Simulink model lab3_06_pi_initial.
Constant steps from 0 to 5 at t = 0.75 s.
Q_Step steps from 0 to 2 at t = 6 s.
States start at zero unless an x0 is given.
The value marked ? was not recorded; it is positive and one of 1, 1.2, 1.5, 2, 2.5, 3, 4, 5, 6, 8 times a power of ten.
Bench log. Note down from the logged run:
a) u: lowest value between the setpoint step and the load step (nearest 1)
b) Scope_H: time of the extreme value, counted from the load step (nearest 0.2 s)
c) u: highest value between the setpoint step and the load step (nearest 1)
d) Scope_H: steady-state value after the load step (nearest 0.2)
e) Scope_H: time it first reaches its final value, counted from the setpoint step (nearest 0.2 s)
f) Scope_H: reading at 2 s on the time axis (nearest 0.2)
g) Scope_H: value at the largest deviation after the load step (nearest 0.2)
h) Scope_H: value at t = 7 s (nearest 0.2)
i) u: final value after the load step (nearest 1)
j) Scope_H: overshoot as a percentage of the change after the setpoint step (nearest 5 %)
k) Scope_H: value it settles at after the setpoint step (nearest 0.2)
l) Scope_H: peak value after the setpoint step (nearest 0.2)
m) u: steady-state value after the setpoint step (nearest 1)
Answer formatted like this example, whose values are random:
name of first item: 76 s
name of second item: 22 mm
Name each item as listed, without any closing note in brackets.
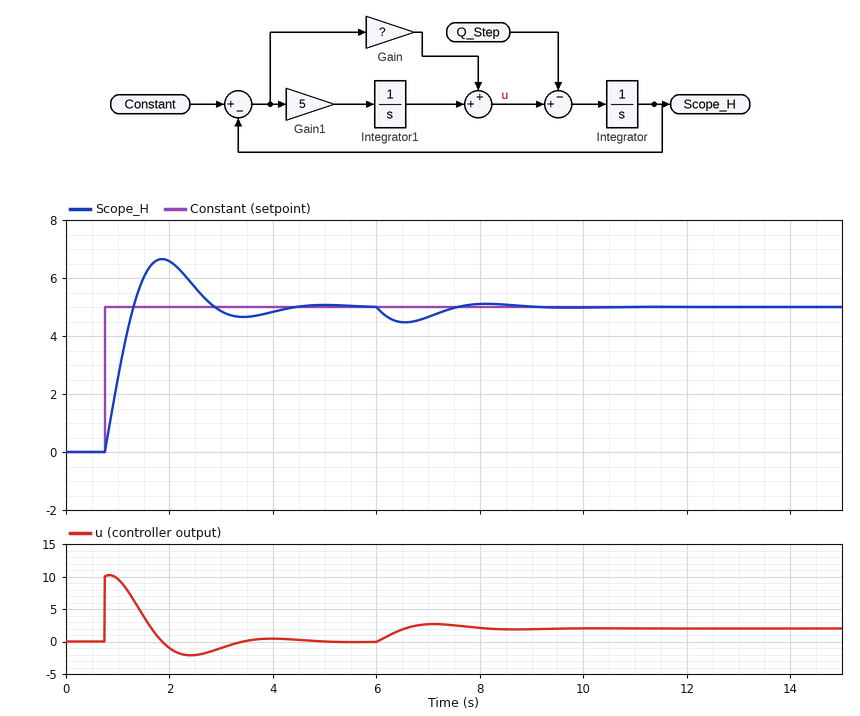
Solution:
u: lowest value between the setpoint step and the load step: -2
Scope_H: time of the extreme value, counted from the load step: 0.6 s
u: highest value between the setpoint step and the load step: 10
Scope_H: steady-state value after the load step: 5.0
Scope_H: time it first reaches its final value, counted from the setpoint step: 0.6 s
Scope_H: reading at 2 s on the time axis: 6.6
Scope_H: value at the largest deviation after the load step: 4.4
Scope_H: value at t = 7 s: 4.6
u: final value after the load step: 2
Scope_H: overshoot as a percentage of the change after the setpoint step: 35 %
Scope_H: value it settles at after the setpoint step: 5.0
Scope_H: peak value after the setpoint step: 6.6
u: steady-state value after the setpoint step: 0
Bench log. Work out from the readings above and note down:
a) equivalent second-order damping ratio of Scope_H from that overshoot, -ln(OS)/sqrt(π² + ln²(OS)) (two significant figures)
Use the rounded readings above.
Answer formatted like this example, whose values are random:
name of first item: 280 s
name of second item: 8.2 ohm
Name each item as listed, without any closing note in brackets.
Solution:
equivalent second-order damping ratio of Scope_H from that overshoot, -ln(OS)/sqrt(π² + ln²(OS)): 0.32
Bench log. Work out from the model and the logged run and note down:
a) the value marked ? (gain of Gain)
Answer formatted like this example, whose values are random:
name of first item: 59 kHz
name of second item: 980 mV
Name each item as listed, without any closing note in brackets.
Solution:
the value marked ?: 2
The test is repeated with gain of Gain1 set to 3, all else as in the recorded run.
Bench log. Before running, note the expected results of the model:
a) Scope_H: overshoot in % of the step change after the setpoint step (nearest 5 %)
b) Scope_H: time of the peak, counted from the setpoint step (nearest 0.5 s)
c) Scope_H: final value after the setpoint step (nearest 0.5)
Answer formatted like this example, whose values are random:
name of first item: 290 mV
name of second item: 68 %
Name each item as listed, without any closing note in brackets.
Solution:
Scope_H: overshoot in % of the step change after the setpoint step: 25 %
Scope_H: time of the peak, counted from the setpoint step: 1.5 s
Scope_H: final value after the setpoint step: 5.0
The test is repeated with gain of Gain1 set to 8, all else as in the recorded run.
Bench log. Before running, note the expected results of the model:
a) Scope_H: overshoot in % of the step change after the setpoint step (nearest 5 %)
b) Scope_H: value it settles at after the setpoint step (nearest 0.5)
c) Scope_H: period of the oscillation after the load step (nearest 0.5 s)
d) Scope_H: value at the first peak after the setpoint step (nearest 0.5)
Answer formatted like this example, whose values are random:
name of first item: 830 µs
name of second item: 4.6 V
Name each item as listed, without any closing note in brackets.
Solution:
Scope_H: overshoot in % of the step change after the setpoint step: 40 %
Scope_H: value it settles at after the setpoint step: 5.0
Scope_H: period of the oscillation after the load step: 2.5 s
Scope_H: value at the first peak after the setpoint step: 7.0
